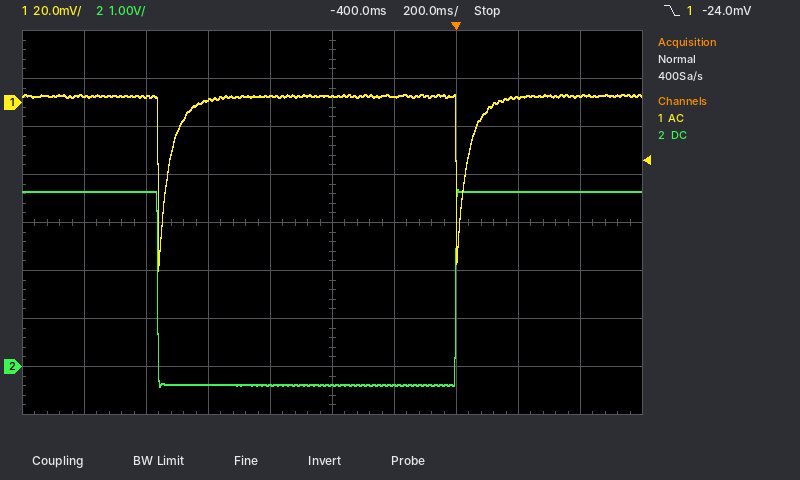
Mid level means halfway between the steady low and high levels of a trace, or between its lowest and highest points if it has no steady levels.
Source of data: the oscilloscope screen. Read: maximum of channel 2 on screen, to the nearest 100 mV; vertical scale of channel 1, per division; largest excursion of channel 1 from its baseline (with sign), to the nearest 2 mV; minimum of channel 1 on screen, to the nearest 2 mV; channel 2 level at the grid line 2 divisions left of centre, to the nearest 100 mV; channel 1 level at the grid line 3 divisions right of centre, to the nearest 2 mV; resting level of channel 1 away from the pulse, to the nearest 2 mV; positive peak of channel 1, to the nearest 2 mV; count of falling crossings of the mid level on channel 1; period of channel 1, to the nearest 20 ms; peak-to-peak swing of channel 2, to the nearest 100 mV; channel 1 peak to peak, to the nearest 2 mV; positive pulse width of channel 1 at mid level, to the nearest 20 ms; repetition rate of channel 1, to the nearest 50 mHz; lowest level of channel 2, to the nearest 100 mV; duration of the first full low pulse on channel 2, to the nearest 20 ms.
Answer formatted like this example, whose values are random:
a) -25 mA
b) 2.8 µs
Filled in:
a) 3.7 V
b) 20 mV
c) -72 mV
d) -70 mV
e) -400 mV
f) 2 mV
g) 2 mV
h) 4 mV
i) 2
j) 960 ms
k) 4.1 V
l) 74 mV
m) 940 ms
n) 1.05 Hz
o) -400 mV
p) 960 ms
